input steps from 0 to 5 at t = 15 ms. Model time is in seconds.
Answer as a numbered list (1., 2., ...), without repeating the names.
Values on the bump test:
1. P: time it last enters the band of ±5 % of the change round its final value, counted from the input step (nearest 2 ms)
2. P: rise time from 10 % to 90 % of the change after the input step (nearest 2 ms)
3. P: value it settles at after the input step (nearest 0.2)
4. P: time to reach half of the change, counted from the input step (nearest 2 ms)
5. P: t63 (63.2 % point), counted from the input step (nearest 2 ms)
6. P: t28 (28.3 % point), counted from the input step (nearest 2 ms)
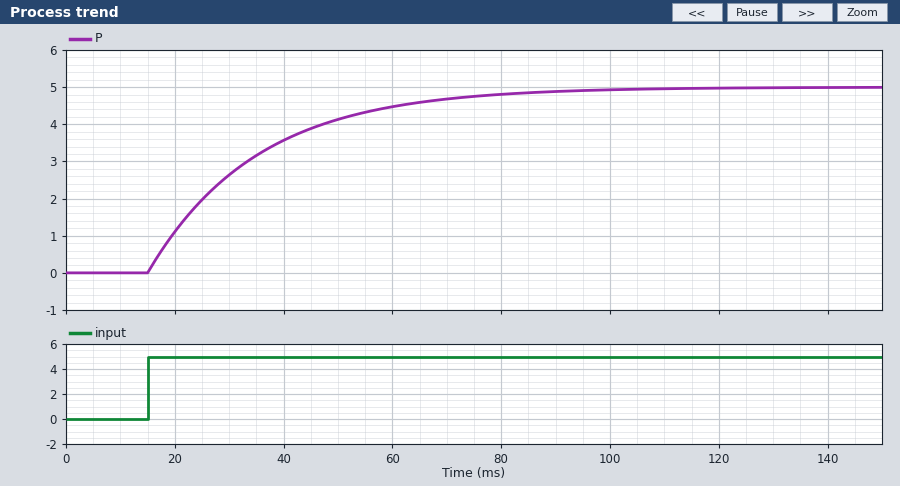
1. 60 ms
2. 44 ms
3. 5.0
4. 14 ms
5. 20 ms
6. 6 ms
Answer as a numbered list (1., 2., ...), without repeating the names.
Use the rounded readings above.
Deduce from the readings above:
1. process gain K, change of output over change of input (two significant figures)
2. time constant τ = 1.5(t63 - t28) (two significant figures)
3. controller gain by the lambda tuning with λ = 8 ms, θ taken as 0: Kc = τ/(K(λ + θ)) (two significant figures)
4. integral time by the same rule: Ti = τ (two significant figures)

1. 1.0
2. 21 ms
3. 2.6
4. 21 ms
